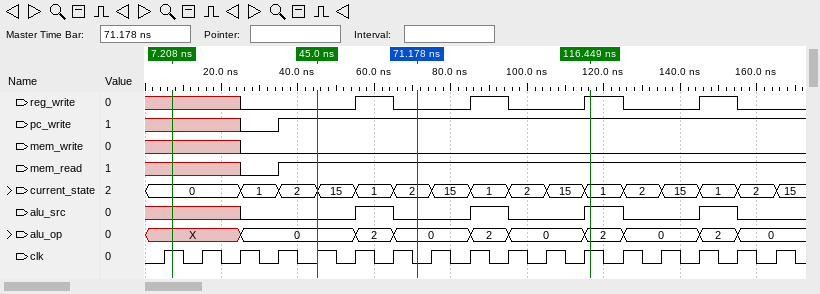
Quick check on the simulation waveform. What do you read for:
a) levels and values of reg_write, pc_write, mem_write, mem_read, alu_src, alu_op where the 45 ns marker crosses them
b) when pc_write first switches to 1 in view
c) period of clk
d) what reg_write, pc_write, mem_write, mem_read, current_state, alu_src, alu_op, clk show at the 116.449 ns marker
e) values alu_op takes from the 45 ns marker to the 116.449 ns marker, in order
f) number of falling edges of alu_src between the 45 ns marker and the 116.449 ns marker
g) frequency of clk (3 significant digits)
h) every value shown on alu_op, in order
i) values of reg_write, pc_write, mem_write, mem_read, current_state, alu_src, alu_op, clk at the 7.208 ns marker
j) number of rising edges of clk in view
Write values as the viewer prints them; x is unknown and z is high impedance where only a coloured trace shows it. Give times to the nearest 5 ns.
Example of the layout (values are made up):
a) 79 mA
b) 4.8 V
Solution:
a) reg_write=0, pc_write=1, mem_write=0, mem_read=1, alu_src=0, alu_op=0
b) 35 ns
c) 10 ns
d) reg_write=1, pc_write=1, mem_write=0, mem_read=1, current_state=1, alu_src=1, alu_op=2, clk=1
e) 0, 2, 0, 2, 0, 2
f) 2
g) 100 MHz
h) X, 0, 2, 0, 2, 0, 2, 0, 2, 0
i) reg_write=x, pc_write=x, mem_write=x, mem_read=x, current_state=0, alu_src=x, alu_op=X, clk=1
j) 17
